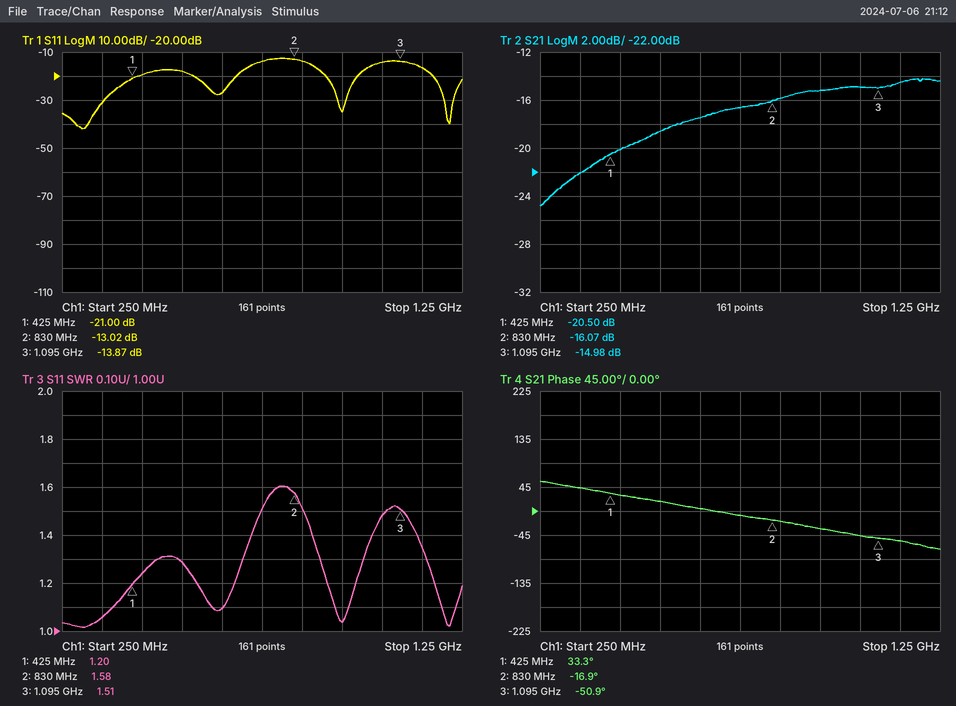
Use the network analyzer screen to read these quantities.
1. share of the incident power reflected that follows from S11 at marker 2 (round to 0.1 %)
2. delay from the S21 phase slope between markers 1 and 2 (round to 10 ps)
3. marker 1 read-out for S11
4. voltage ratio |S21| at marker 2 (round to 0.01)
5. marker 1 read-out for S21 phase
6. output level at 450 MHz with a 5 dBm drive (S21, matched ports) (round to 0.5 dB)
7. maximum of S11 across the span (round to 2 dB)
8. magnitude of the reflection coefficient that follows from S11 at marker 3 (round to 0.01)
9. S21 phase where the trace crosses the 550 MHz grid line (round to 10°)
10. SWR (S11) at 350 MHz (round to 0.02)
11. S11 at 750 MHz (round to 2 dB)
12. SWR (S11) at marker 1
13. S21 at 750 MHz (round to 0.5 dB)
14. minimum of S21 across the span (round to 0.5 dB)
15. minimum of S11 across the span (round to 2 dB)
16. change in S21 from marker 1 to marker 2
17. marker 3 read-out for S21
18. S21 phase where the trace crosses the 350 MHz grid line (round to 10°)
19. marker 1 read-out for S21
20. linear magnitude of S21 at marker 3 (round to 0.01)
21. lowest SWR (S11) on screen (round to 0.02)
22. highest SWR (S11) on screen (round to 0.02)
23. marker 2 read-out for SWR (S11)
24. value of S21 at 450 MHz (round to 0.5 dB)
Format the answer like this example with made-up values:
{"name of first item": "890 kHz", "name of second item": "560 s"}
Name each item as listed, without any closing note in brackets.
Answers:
{"share of the incident power reflected that follows from S11 at marker 2": "5.0 %", "delay from the S21 phase slope between markers 1 and 2": "340 ps", "marker 1 read-out for S11": "-21.00 dB", "voltage ratio |S21| at marker 2": "0.16", "marker 1 read-out for S21 phase": "33.3°", "output level at 450 MHz with a 5 dBm drive (S21, matched ports)": "-15.0 dBm", "maximum of S11 across the span": "-12 dB", "magnitude of the reflection coefficient that follows from S11 at marker 3": "0.20", "S21 phase where the trace crosses the 550 MHz grid line": "20°", "SWR (S11) at 350 MHz": "1.06", "S11 at 750 MHz": "-14 dB", "SWR (S11) at marker 1": "1.20", "S21 at 750 MHz": "-16.5 dB", "minimum of S21 across the span": "-25.0 dB", "minimum of S11 across the span": "-42 dB", "change in S21 from marker 1 to marker 2": "4.43 dB", "marker 3 read-out for S21": "-14.98 dB", "S21 phase where the trace crosses the 350 MHz grid line": "40°", "marker 1 read-out for S21": "-20.50 dB", "linear magnitude of S21 at marker 3": "0.18", "lowest SWR (S11) on screen": "1.02", "highest SWR (S11) on screen": "1.60", "marker 2 read-out for SWR": "1.58", "value of S21 at 450 MHz": "-20.0 dB"}
